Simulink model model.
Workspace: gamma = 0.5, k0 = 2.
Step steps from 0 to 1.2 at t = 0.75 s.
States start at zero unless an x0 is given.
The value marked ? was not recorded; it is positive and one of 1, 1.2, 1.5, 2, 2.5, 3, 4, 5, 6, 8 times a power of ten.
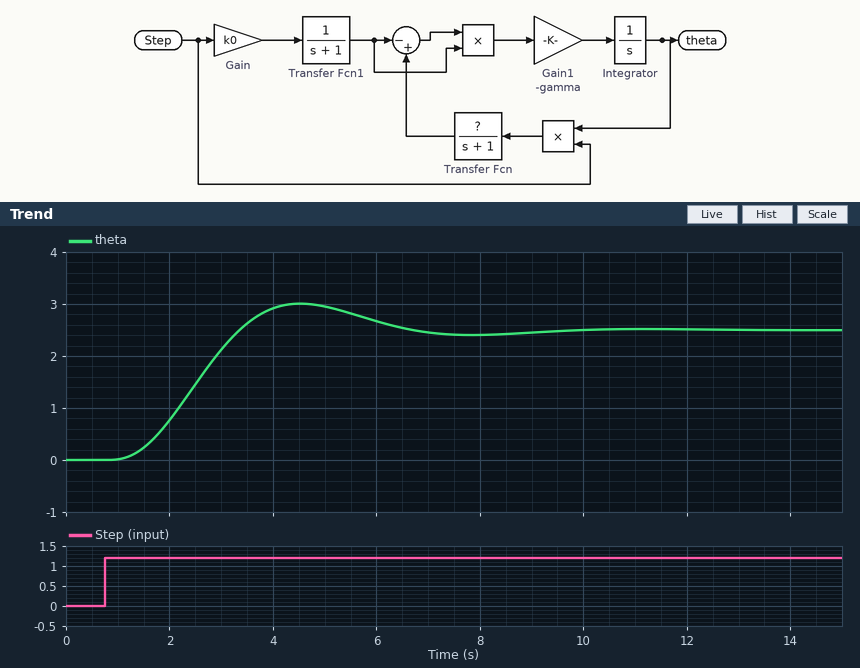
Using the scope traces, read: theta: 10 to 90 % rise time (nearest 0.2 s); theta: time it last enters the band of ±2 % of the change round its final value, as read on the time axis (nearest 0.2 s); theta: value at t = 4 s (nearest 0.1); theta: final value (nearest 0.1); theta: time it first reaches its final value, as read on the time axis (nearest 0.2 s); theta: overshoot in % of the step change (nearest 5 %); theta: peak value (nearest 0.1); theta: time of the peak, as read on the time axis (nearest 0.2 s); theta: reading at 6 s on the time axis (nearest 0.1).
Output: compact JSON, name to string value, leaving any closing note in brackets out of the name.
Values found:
{"theta: 10 to 90 % rise time": "1.6 s", "theta: time it last enters the band of ±2 % of the change round its final value, as read on the time axis": "9.0 s", "theta: value at t = 4 s": "2.9", "theta: final value": "2.5", "theta: time it first reaches its final value, as read on the time axis": "3.4 s", "theta: overshoot in % of the step change": "20 %", "theta: peak value": "3.0", "theta: time of the peak, as read on the time axis": "4.6 s", "theta: reading at 6 s on the time axis": "2.7"}
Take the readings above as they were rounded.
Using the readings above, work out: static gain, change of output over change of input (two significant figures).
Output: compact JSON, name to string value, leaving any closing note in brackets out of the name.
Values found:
{"static gain, change of output over change of input": "2.1"}
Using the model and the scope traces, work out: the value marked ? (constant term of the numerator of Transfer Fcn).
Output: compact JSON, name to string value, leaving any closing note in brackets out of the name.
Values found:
{"the value marked ?": "0.8"}
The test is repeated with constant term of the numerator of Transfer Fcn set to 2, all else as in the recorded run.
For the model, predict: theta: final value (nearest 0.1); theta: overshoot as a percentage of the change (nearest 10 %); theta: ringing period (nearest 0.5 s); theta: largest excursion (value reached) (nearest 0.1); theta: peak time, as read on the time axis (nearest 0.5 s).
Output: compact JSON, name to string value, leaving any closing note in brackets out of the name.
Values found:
{"theta: final value": "1.0", "theta: overshoot as a percentage of the change": "40 %", "theta: ringing period": "4.0 s", "theta: largest excursion (value reached)": "1.4", "theta: peak time, as read on the time axis": "3.0 s"}
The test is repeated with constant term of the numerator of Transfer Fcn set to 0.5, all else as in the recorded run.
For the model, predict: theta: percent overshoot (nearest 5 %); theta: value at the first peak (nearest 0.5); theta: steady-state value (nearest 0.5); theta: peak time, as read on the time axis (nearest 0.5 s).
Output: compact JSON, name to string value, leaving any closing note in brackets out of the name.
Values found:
{"theta: percent overshoot": "10 %", "theta: value at the first peak": "4.5", "theta: steady-state value": "4.0", "theta: peak time, as read on the time axis": "6.0 s"}
